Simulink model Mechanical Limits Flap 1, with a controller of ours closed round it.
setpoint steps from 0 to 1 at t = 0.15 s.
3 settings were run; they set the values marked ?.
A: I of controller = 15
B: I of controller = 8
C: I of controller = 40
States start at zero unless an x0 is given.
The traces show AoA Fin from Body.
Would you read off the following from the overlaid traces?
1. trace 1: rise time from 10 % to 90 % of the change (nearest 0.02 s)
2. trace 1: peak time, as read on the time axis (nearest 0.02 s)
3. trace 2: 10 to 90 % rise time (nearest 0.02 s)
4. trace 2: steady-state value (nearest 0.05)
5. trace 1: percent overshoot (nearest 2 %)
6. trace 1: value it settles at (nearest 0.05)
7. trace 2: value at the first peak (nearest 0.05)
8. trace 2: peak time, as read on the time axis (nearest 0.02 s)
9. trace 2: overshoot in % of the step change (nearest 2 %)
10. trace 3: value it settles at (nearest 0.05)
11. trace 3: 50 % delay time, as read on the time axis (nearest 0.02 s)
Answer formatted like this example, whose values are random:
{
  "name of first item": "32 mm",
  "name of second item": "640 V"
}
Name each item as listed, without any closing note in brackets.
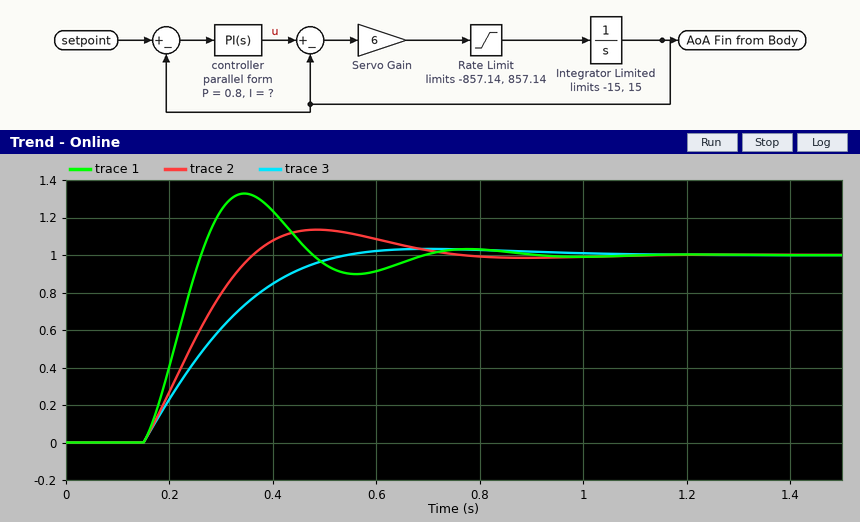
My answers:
{
  "trace 1: rise time from 10 % to 90 % of the change": "0.08 s",
  "trace 1: peak time, as read on the time axis": "0.34 s",
  "trace 2: 10 to 90 % rise time": "0.16 s",
  "trace 2: steady-state value": "1.00",
  "trace 1: percent overshoot": "32 %",
  "trace 1: value it settles at": "1.00",
  "trace 2: value at the first peak": "1.15",
  "trace 2: peak time, as read on the time axis": "0.48 s",
  "trace 2: overshoot in % of the step change": "14 %",
  "trace 3: value it settles at": "1.00",
  "trace 3: 50 % delay time, as read on the time axis": "0.26 s"
}
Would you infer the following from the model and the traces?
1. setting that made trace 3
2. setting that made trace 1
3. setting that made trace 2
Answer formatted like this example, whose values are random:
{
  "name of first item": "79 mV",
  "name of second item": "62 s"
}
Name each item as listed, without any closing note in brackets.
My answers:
{
  "setting that made trace 3": "B",
  "setting that made trace 1": "C",
  "setting that made trace 2": "A"
}
